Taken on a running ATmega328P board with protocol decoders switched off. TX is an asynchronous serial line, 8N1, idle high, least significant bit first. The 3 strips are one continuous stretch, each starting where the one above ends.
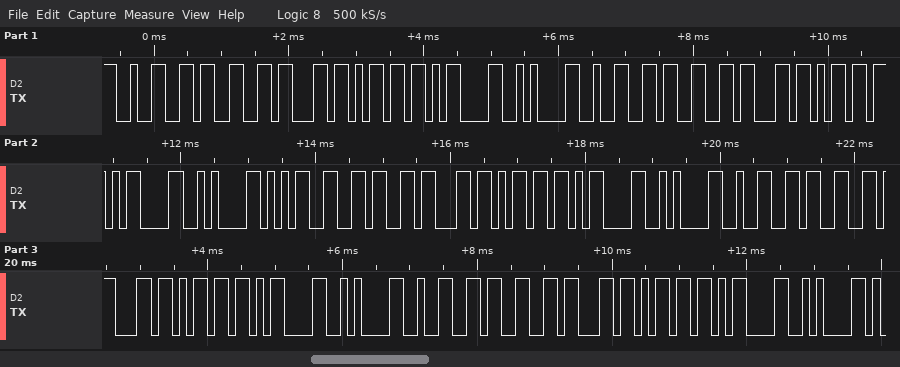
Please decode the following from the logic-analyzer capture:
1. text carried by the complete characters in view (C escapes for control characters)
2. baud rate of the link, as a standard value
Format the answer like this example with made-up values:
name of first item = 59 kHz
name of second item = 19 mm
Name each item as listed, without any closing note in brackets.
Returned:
text carried by the complete characters in view = "23cm\r\n23cm\r\n56cm\r\n23cm\r\n23cm\r\n"
baud rate of the link, as a standard value = 9600 baud
